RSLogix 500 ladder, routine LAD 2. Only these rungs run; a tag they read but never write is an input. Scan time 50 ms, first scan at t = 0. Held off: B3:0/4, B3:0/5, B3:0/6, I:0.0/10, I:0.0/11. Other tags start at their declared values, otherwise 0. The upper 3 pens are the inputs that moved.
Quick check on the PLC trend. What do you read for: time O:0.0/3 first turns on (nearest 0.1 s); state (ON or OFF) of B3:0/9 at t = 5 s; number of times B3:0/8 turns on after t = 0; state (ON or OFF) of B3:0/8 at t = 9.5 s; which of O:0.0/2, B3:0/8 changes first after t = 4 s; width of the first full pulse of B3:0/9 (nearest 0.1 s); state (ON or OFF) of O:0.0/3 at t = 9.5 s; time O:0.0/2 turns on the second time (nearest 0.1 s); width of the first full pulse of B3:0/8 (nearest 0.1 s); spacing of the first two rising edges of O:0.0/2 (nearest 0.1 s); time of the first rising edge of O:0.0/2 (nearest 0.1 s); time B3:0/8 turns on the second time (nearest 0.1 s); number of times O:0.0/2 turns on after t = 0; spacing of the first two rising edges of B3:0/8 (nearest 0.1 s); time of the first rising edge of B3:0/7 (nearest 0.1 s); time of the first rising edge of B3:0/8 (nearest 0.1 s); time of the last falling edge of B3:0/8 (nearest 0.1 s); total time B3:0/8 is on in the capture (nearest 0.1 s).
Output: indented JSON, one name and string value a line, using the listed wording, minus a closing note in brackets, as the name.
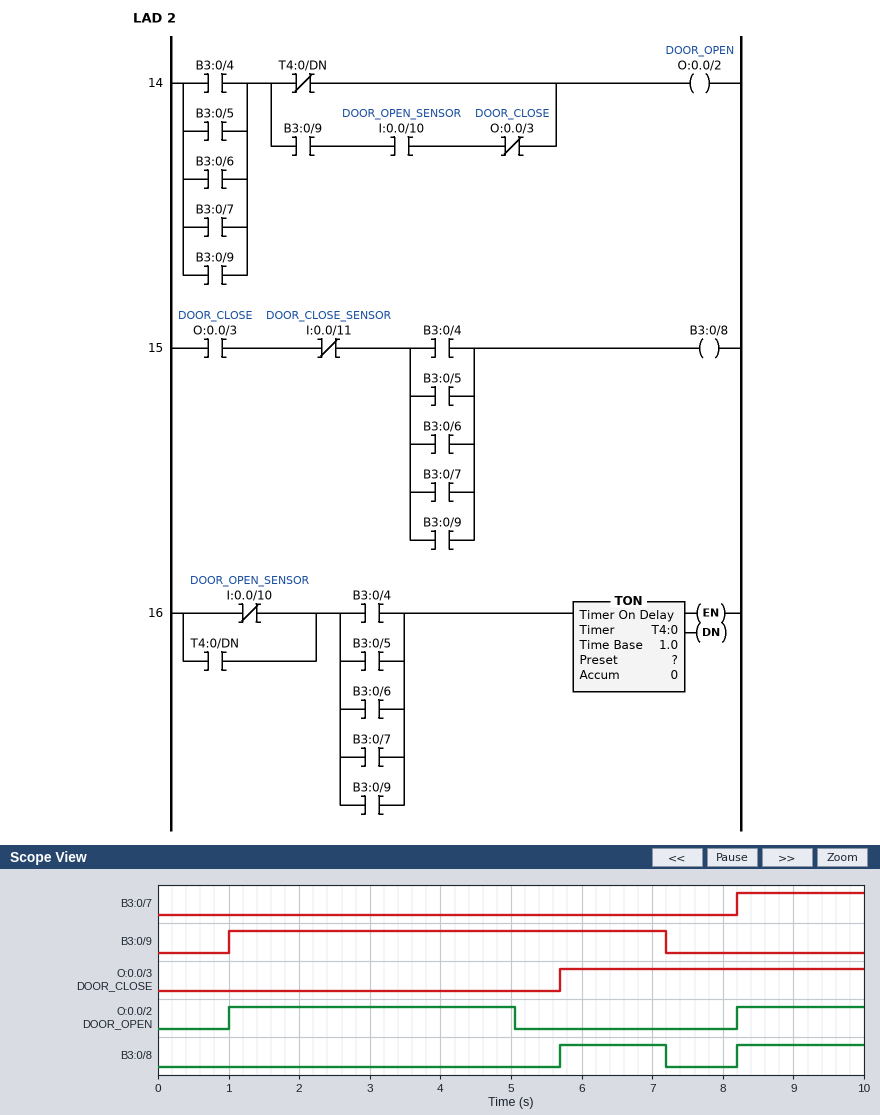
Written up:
{
  "time O:0.0/3 first turns on": "5.7 s",
  "state (ON or OFF) of B3:0/9 at t = 5 s": "ON",
  "number of times B3:0/8 turns on after t = 0": "2",
  "state (ON or OFF) of B3:0/8 at t = 9.5 s": "ON",
  "which of O:0.0/2, B3:0/8 changes first after t = 4 s": "O:0.0/2",
  "width of the first full pulse of B3:0/9": "6.2 s",
  "state (ON or OFF) of O:0.0/3 at t = 9.5 s": "ON",
  "time O:0.0/2 turns on the second time": "8.2 s",
  "width of the first full pulse of B3:0/8": "1.5 s",
  "spacing of the first two rising edges of O:0.0/2": "7.2 s",
  "time of the first rising edge of O:0.0/2": "1.0 s",
  "time B3:0/8 turns on the second time": "8.2 s",
  "number of times O:0.0/2 turns on after t = 0": "2",
  "spacing of the first two rising edges of B3:0/8": "2.5 s",
  "time of the first rising edge of B3:0/7": "8.2 s",
  "time of the first rising edge of B3:0/8": "5.7 s",
  "time of the last falling edge of B3:0/8": "7.2 s",
  "total time B3:0/8 is on in the capture": "3.3 s"
}
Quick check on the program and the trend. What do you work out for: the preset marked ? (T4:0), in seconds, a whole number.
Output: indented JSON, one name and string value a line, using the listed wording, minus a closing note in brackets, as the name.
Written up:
{
  "the preset marked ? (T4:0), in seconds, a whole number": "4 s"
}
